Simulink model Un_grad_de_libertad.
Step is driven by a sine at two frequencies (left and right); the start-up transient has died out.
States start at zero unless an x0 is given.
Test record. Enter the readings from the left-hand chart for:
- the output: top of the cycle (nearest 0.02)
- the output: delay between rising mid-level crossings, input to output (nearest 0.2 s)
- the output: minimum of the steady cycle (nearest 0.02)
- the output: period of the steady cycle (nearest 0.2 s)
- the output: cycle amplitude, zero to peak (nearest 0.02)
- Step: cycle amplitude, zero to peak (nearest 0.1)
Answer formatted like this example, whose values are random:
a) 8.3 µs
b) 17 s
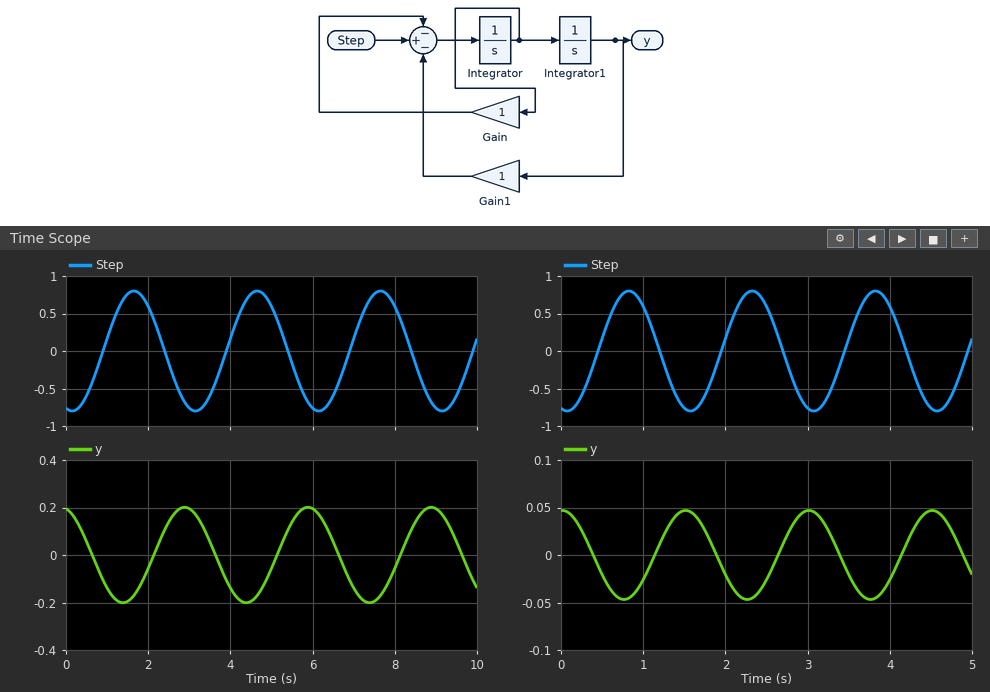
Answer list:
a) 0.20
b) 1.2 s
c) -0.20
d) 3.0 s
e) 0.20
f) 0.8
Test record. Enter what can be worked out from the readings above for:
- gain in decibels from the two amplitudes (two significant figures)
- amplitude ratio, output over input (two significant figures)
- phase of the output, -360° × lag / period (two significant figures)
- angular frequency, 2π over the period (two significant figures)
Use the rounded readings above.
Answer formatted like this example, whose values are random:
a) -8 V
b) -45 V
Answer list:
a) -12 dB
b) 0.25
c) -140°
d) 2.1 rad/s
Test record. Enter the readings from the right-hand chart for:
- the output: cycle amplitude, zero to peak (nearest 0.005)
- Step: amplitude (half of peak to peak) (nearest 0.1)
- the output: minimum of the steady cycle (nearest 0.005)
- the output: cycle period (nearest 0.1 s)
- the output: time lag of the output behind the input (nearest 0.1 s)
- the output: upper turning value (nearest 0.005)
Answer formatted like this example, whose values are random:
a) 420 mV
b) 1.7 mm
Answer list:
a) 0.045
b) 0.8
c) -0.045
d) 1.5 s
e) 0.7 s
f) 0.045
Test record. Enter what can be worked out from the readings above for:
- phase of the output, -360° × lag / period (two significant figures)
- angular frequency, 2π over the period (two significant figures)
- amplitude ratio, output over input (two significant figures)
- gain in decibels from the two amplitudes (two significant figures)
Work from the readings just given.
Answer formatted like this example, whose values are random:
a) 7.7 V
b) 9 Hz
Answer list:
a) -170°
b) 4.2 rad/s
c) 0.056
d) -25 dB
